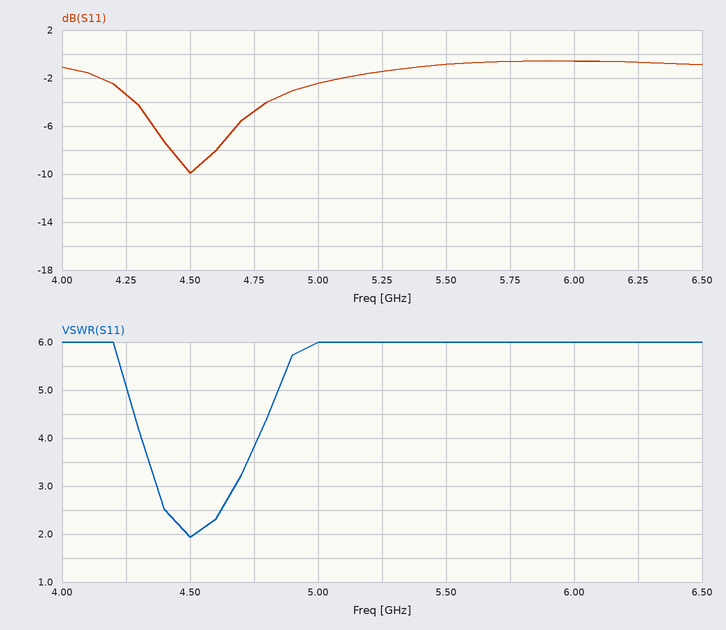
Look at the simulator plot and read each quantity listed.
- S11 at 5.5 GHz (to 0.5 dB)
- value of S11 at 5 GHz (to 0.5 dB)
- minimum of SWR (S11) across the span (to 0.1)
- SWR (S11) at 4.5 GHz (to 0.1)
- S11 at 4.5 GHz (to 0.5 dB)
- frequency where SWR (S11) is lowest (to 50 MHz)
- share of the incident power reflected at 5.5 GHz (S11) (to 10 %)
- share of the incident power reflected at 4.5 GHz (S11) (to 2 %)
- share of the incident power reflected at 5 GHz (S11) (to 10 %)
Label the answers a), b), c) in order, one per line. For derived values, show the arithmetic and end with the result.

a) -1.0 dB
b) -2.5 dB
c) 1.9
d) 1.9
e) -10.0 dB
f) 4.50 GHz
g) 10^(-1/10) ≈ 79.4 %, so 80 % to the nearest 10 %
h) 10^(-10/10) ≈ 10 %
i) 10^(-2.5/10) ≈ 56.2 %, so 60 % to the nearest 10 %
